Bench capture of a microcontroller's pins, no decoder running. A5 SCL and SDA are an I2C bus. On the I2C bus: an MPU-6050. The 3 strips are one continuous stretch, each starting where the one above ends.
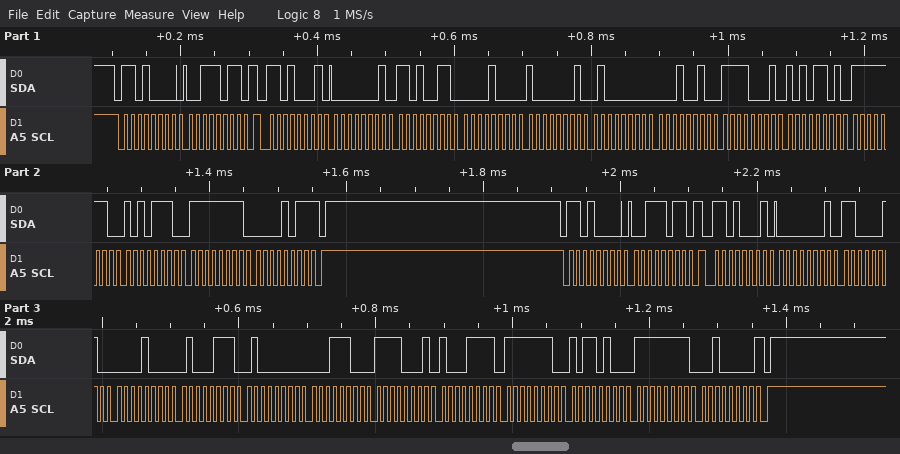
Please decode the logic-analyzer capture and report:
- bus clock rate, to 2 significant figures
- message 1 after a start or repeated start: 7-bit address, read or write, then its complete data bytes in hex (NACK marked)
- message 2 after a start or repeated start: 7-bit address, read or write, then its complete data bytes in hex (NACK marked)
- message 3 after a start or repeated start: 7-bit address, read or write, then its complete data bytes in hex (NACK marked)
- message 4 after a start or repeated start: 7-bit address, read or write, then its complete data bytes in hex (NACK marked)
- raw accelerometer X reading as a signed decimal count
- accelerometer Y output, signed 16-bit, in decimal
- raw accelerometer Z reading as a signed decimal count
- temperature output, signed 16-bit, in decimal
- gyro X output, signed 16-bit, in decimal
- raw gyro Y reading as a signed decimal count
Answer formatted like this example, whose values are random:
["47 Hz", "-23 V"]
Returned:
["100 kHz", "0x68 write: 3B", "0x68 read: 01 D3 08 81 40 12 F1 AD FE AE FF 0B NACK", "0x68 write: 3B", "0x68 read: 01 C2 08 47 40 1C F1 8F FE B4 FF 20 NACK", "467", "2177", "16402", "-3667", "-338", "-245"]
